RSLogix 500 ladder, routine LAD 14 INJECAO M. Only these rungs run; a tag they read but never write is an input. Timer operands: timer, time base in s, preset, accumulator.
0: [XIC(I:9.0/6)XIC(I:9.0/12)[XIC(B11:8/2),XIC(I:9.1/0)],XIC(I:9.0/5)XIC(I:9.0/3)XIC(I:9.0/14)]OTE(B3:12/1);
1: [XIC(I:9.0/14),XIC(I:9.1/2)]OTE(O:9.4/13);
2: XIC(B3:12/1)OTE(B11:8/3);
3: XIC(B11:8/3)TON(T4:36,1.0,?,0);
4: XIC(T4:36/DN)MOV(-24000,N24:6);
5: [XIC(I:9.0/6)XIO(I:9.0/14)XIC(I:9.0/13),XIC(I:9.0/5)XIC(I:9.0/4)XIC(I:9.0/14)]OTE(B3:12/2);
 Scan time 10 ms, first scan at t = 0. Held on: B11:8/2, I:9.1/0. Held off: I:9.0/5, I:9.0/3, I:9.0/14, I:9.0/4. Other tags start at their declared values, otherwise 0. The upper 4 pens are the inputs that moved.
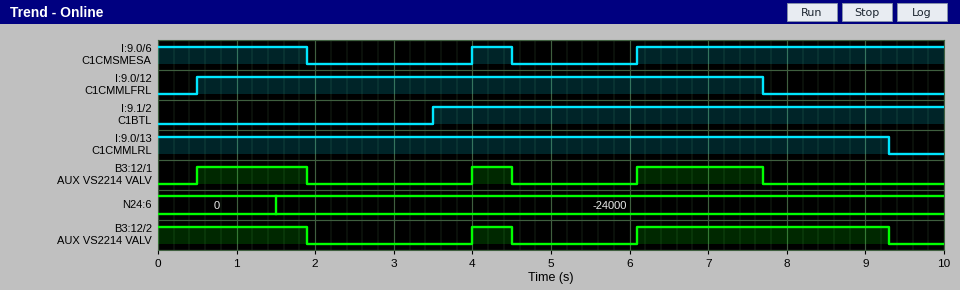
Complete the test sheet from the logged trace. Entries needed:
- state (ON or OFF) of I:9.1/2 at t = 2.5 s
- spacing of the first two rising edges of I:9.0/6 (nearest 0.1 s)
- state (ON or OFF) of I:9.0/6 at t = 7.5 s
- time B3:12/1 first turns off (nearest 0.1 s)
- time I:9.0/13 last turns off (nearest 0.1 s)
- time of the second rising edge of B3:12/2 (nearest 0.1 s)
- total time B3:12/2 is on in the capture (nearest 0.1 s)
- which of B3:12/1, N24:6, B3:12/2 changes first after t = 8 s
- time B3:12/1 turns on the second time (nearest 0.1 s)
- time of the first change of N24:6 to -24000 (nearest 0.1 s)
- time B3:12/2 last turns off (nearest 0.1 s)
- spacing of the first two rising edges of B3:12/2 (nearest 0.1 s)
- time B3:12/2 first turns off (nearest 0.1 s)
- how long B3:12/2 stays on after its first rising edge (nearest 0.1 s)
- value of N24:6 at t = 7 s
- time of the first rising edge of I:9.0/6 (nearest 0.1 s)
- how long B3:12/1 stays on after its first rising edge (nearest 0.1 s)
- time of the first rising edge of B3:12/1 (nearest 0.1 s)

OFF
2.1 s
ON
1.9 s
9.3 s
6.1 s
5.6 s
B3:12/2
4.0 s
1.5 s
9.3 s
2.1 s
1.9 s
0.5 s
-24000
4.0 s
1.4 s
0.5 s
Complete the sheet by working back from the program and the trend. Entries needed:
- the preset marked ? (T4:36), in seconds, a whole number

1 s
